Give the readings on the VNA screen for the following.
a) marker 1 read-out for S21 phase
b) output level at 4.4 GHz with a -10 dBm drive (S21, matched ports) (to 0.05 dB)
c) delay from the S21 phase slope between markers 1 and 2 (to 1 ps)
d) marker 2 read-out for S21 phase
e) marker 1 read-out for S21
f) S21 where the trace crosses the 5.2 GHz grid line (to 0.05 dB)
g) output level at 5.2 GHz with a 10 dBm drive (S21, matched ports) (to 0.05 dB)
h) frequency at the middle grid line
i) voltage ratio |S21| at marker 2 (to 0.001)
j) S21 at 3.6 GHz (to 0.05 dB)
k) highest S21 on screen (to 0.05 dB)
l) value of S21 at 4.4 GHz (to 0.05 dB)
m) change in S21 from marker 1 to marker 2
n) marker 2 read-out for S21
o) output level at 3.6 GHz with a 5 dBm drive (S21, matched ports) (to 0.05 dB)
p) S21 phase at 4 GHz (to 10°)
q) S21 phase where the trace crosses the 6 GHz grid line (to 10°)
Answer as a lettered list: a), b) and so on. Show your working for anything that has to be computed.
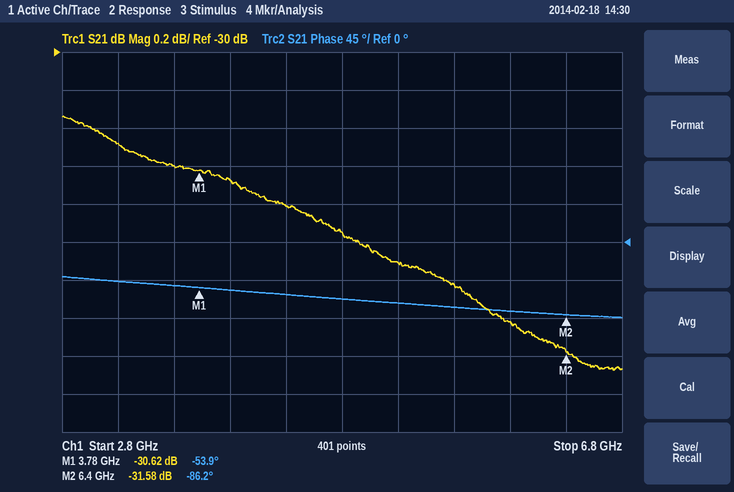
a) -53.9°
b) -10 dBm + (-30.80 dB) = -40.80 dBm
c) −(-86.2° − (-53.9°))/(360° × 2.62 GHz) ≈ 34 ps
d) -86.2°
e) -30.62 dB
f) -31.10 dB
g) 10 dBm + (-31.10 dB) = -21.10 dBm
h) 4.8 GHz
i) 10^(-31.58/20) ≈ 0.026
j) -30.60 dB
k) -30.35 dB
l) -30.80 dB
m) -31.58 − (-30.62) = -0.96 dB
n) -31.58 dB
o) 5 dBm + (-30.60 dB) = -25.60 dBm
p) -60°
q) -80°
